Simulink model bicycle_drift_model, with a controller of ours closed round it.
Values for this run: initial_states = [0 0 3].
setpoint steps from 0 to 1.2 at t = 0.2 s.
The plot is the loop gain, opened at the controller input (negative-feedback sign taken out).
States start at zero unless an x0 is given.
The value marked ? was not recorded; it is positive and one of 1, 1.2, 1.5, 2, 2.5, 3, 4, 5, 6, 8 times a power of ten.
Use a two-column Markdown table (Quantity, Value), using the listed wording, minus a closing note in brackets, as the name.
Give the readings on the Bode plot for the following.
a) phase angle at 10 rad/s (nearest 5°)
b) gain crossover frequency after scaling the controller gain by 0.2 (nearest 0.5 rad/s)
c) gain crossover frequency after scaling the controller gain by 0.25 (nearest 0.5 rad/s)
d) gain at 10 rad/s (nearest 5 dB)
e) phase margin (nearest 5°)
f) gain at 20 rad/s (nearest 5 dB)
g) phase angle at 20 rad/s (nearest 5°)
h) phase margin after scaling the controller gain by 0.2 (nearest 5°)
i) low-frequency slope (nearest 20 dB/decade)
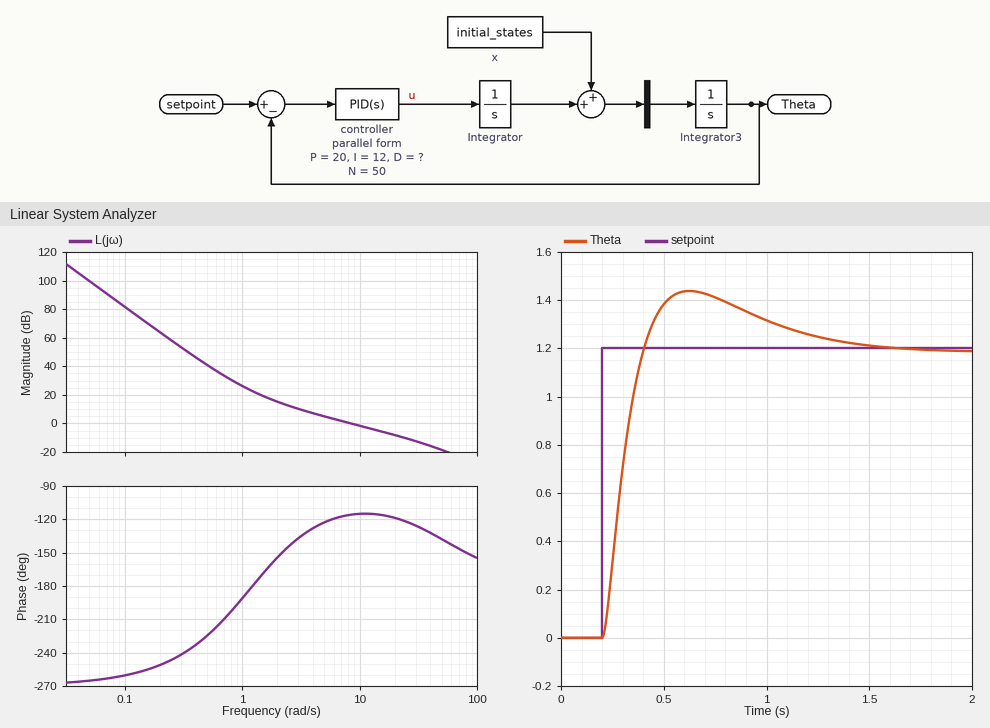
| Quantity | Value |
|---|---|
| phase angle at 10 rad/s | -115° |
| gain crossover frequency after scaling the controller gain by 0.2 | 2.0 rad/s |
| gain crossover frequency after scaling the controller gain by 0.25 | 2.5 rad/s |
| gain at 10 rad/s | 0 dB |
| phase margin | 65° |
| gain at 20 rad/s | -10 dB |
| phase angle at 20 rad/s | -120° |
| phase margin after scaling the controller gain by 0.2 | 30° |
| low-frequency slope | -60 dB/decade |
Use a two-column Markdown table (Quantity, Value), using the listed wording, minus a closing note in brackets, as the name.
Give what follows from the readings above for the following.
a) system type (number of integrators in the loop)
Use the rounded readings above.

| Quantity | Value |
|---|---|
| system type | 3 |
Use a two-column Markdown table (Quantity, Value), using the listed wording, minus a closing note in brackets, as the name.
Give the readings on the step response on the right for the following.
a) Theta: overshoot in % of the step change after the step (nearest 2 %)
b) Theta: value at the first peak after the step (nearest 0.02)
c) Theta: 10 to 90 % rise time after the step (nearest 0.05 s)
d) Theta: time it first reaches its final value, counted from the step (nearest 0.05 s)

| Quantity | Value |
|---|---|
| Theta: overshoot in % of the step change after the step | 20 % |
| Theta: value at the first peak after the step | 1.44 |
| Theta: 10 to 90 % rise time after the step | 0.15 s |
| Theta: time it first reaches its final value, counted from the step | 0.20 s |
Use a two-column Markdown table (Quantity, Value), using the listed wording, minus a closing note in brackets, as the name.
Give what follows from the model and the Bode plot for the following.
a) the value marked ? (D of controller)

| Quantity | Value |
|---|---|
| the value marked ? | 8 |
